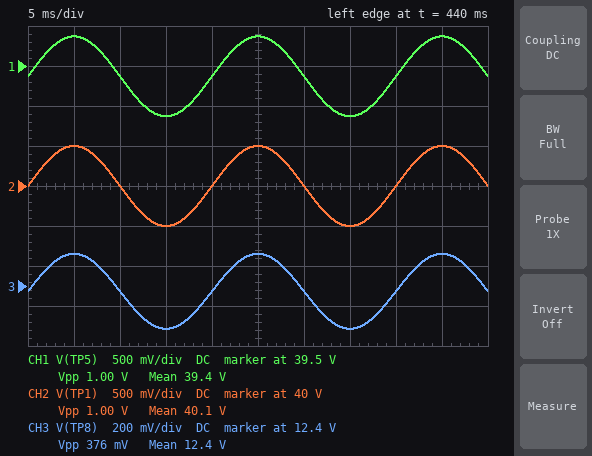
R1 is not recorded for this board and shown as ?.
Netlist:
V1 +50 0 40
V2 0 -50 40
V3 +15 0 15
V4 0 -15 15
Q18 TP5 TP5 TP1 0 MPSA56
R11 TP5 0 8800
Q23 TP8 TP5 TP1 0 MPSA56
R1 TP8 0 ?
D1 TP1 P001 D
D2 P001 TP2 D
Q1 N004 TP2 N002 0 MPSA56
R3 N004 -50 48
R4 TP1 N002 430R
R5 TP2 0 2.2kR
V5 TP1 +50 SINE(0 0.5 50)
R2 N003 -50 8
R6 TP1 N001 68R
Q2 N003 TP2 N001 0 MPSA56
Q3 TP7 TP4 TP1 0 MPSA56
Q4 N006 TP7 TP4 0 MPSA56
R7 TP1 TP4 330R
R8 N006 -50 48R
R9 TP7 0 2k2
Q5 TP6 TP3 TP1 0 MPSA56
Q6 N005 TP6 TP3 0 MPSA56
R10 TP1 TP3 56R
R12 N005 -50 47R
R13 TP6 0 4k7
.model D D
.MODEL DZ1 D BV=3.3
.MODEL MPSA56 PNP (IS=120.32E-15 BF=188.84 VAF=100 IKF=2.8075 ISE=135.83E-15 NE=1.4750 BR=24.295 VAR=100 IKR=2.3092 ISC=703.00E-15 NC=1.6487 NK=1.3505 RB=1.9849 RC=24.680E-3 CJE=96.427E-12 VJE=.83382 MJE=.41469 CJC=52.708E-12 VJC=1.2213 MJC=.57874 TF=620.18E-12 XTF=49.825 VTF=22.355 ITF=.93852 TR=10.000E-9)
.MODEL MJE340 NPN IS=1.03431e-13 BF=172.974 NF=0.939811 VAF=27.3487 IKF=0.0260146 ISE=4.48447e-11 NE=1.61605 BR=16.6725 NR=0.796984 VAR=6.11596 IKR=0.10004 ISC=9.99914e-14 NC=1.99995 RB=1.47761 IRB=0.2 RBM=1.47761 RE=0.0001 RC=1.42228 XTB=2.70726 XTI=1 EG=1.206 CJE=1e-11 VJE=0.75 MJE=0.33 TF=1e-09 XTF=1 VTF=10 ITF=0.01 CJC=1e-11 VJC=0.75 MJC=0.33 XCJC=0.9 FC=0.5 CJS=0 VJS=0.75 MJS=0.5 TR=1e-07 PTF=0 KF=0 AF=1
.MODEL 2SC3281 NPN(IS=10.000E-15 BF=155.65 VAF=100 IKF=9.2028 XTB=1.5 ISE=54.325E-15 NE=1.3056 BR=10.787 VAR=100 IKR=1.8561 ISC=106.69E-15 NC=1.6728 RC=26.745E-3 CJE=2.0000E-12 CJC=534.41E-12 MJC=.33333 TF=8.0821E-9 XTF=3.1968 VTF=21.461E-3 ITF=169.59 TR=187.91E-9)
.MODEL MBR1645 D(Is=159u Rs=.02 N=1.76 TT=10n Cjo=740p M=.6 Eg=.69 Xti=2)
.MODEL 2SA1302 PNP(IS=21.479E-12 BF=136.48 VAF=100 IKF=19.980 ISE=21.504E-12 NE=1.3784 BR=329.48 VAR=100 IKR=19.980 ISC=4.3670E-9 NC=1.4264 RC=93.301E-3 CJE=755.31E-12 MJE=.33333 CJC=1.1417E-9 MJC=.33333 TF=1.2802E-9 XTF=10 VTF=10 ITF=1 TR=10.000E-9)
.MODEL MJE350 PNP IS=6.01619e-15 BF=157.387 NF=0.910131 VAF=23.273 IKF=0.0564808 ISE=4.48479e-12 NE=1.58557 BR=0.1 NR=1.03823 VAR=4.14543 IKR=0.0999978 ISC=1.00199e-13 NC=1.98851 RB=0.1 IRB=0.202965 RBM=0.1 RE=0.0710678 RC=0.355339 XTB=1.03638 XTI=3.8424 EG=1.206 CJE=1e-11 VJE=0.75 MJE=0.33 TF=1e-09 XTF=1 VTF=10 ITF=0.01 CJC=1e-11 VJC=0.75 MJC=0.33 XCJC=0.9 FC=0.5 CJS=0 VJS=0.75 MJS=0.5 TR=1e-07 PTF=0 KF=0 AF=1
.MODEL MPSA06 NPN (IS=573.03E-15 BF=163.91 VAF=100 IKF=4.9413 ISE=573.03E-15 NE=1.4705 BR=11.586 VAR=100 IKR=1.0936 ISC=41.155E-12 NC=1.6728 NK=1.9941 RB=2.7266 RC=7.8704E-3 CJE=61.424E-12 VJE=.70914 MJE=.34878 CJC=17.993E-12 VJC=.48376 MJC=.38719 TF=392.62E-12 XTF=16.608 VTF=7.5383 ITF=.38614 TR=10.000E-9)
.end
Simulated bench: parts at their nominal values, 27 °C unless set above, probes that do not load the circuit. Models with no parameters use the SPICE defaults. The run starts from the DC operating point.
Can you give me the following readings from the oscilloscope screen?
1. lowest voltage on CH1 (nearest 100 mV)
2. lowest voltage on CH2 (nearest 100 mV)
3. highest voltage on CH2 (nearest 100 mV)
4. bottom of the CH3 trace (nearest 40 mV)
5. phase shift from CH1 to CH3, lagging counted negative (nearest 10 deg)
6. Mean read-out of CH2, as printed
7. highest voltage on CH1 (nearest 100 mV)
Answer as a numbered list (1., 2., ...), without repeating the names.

1. 38.9 V
2. 39.5 V
3. 40.5 V
4. 12.20 V
5. 0 deg
6. 40.1 V
7. 39.9 V
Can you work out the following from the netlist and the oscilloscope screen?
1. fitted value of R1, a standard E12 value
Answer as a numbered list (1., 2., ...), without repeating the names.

1. 2.2 kΩ
